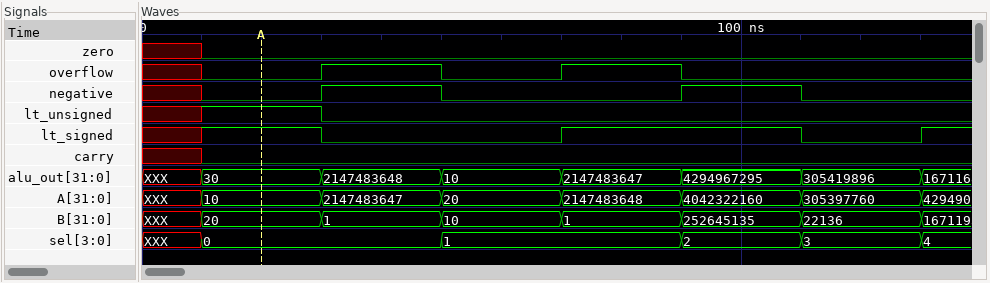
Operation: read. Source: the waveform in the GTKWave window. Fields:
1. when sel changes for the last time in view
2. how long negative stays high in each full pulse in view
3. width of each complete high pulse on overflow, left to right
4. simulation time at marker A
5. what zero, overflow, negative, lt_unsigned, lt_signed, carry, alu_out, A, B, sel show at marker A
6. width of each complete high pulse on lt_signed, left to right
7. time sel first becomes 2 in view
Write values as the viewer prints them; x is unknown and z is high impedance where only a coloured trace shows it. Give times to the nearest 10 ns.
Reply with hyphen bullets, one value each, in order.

- 130 ns
- 20 ns, 20 ns
- 20 ns, 20 ns
- 20 ns
- zero=0, overflow=0, negative=0, lt_unsigned=1, lt_signed=1, carry=0, alu_out=30, A=10, B=20, sel=0
- 40 ns
- 90 ns
